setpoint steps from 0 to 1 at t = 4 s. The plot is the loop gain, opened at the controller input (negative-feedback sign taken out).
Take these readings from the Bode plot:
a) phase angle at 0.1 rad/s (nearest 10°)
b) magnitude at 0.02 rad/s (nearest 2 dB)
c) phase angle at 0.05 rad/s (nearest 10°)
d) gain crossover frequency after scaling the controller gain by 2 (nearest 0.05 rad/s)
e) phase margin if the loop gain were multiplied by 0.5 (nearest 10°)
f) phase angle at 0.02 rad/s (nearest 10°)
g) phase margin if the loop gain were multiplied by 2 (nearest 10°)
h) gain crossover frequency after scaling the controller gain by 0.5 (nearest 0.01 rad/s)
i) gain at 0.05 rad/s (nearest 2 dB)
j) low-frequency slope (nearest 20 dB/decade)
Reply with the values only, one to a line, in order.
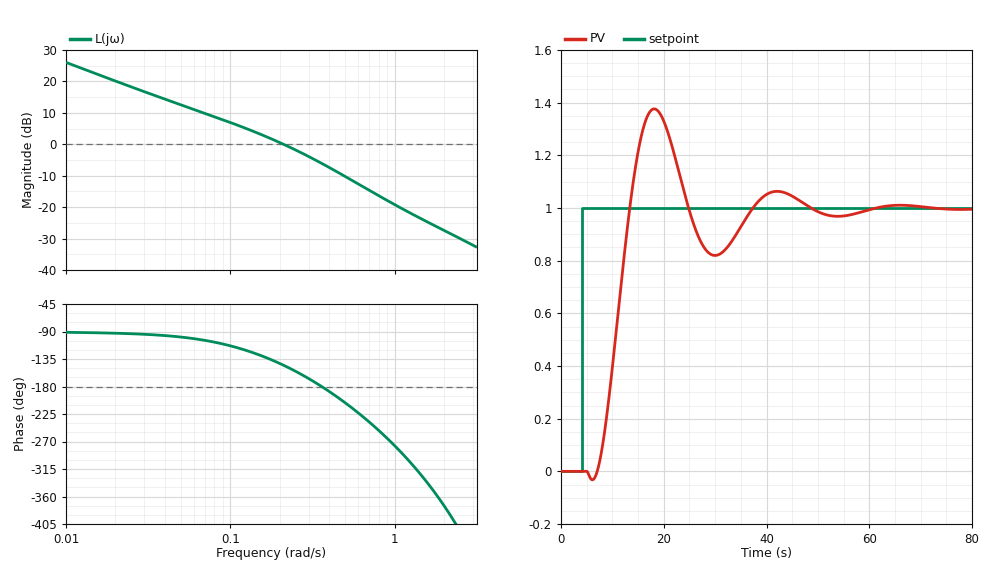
-110°
20 dB
-100°
0.35 rad/s
60°
-90°
0°
0.11 rad/s
12 dB
-20 dB/decade
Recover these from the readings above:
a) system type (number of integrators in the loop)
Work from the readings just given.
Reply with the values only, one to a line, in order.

1
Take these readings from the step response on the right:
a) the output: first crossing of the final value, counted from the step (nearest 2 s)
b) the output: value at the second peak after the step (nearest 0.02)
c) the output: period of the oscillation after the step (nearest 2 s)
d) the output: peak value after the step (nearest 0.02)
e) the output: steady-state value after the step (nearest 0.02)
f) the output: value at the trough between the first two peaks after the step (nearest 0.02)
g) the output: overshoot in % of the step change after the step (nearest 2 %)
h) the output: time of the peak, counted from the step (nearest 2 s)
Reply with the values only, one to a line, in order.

10 s
1.06
24 s
1.38
1.00
0.82
38 %
14 s
